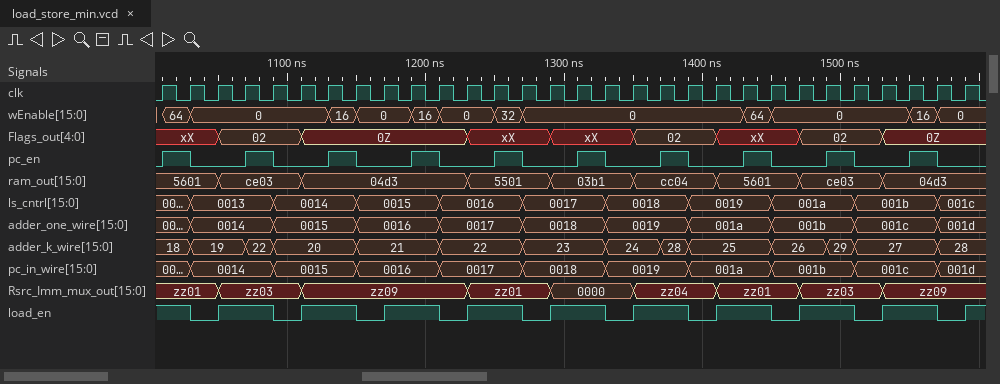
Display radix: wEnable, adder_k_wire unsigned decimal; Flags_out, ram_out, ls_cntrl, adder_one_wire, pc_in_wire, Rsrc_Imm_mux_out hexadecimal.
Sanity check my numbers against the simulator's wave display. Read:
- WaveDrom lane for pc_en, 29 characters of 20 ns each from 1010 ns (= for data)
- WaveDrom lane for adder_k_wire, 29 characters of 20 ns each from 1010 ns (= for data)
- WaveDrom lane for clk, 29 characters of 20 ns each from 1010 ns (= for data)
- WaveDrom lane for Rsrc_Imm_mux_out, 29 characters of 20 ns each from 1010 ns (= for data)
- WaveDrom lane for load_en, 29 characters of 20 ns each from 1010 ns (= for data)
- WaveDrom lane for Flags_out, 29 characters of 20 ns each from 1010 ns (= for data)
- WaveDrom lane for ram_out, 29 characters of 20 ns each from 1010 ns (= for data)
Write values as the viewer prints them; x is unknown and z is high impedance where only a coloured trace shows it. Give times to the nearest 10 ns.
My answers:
{name: 'pc_en', wave: '10.10.10.10.10.10.10.10.10.10'}
{name: 'adder_k_wire', wave: '==.==..=..=..=..=.==..=.==..=', data: '18 19 22 20 21 22 23 24 28 25 26 29 27 28'}
{name: 'clk', wave: 'p............................'}
{name: 'Rsrc_Imm_mux_out', wave: '=.=..=.....=..=..=..=..=..=..', data: 'zz01 zz03 zz09 zz01 0000 zz04 zz01 zz03 zz09'}
{name: 'load_en', wave: '101.01.01.01.01.01.01.01.01.0'}
{name: 'Flags_out', wave: '=.=..=.....=..=..=..=..=..=..', data: 'xX 02 0Z xX xX 02 xX 02 0Z'}
{name: 'ram_out', wave: '=.=..=.....=..=..=..=..=..=..', data: '5601 ce03 04d3 5501 03b1 cc04 5601 ce03 04d3'}
